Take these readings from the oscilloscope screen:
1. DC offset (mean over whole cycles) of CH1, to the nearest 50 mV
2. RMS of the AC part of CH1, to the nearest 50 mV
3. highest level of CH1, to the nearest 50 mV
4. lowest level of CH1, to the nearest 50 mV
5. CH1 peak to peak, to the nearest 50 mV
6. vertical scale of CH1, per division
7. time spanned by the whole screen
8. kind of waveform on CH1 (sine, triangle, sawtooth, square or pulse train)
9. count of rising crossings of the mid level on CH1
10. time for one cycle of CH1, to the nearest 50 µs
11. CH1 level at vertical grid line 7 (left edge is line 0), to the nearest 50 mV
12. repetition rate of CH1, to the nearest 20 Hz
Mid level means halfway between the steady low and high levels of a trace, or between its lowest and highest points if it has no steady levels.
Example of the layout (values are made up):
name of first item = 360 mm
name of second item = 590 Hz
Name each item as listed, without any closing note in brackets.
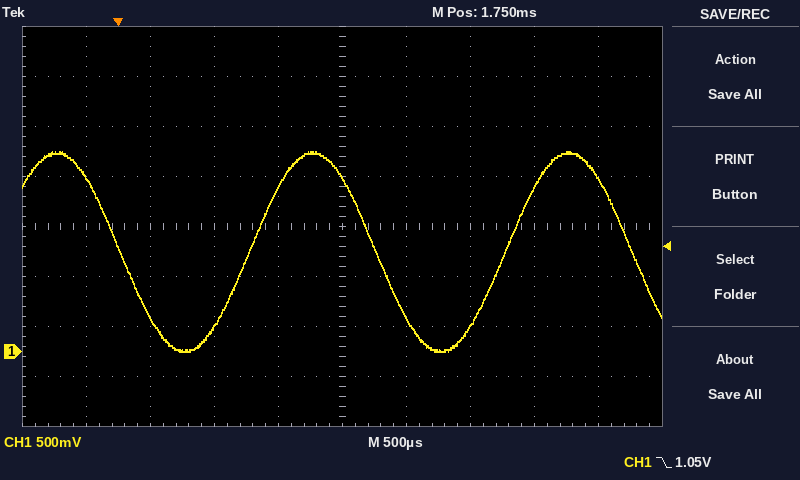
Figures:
DC offset (mean over whole cycles) of CH1, to the nearest 50 mV = 1.00 V
RMS of the AC part of CH1, to the nearest 50 mV = 700 mV
highest level of CH1, to the nearest 50 mV = 2.00 V
lowest level of CH1, to the nearest 50 mV = 0 mV
CH1 peak to peak, to the nearest 50 mV = 2.00 V
vertical scale of CH1, per division = 500 mV
time spanned by the whole screen = 5 ms
kind of waveform on CH1 = sine
count of rising crossings of the mid level on CH1 = 2
time for one cycle of CH1, to the nearest 50 µs = 2.00 ms
CH1 level at vertical grid line 7 (left edge is line 0), to the nearest 50 mV = 250 mV
repetition rate of CH1, to the nearest 20 Hz = 500 Hz
